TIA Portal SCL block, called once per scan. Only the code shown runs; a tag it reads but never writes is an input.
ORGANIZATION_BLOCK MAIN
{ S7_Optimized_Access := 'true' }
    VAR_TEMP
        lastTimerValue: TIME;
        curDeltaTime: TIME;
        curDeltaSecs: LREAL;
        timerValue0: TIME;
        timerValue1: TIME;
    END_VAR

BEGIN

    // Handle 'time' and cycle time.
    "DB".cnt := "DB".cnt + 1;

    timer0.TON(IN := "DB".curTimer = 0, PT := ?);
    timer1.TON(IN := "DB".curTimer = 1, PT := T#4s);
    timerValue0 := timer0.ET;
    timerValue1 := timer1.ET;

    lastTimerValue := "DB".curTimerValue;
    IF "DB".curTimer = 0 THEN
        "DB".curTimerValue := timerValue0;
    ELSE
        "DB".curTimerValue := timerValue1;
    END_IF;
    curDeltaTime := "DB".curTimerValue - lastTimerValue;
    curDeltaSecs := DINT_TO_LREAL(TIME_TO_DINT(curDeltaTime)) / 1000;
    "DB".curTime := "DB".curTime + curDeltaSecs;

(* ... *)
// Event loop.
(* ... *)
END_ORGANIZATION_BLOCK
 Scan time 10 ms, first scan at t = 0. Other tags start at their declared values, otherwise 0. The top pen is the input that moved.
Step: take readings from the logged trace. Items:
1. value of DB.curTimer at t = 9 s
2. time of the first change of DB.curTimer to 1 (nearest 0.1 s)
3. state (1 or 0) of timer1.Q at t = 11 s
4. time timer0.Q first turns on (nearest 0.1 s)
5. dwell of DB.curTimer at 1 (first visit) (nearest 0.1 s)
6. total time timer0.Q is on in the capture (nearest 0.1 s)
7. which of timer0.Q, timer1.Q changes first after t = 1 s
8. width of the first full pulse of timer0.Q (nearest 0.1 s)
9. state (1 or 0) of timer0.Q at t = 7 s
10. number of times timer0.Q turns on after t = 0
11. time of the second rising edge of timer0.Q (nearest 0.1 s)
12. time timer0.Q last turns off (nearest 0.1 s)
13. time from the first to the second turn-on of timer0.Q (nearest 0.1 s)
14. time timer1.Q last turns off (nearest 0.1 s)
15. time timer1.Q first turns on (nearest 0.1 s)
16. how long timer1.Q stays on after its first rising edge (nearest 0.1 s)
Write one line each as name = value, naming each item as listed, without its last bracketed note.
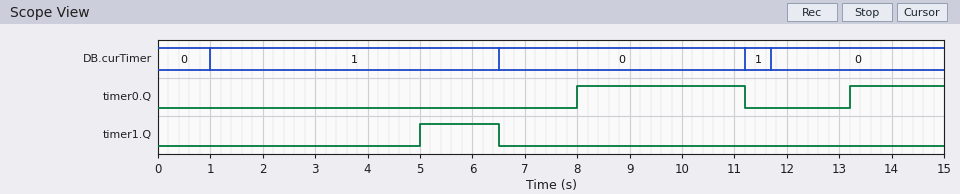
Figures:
value of DB.curTimer at t = 9 s = 0
time of the first change of DB.curTimer to 1 = 1.0 s
state (1 or 0) of timer1.Q at t = 11 s = 0
time timer0.Q first turns on = 8.0 s
dwell of DB.curTimer at 1 (first visit) = 5.5 s
total time timer0.Q is on in the capture = 5.0 s
which of timer0.Q, timer1.Q changes first after t = 1 s = timer1.Q
width of the first full pulse of timer0.Q = 3.2 s
state (1 or 0) of timer0.Q at t = 7 s = 0
number of times timer0.Q turns on after t = 0 = 2
time of the second rising edge of timer0.Q = 13.2 s
time timer0.Q last turns off = 11.2 s
time from the first to the second turn-on of timer0.Q = 5.2 s
time timer1.Q last turns off = 6.5 s
time timer1.Q first turns on = 5.0 s
how long timer1.Q stays on after its first rising edge = 1.5 s
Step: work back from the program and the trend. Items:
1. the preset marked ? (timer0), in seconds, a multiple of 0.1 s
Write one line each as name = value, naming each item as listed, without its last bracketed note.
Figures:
the preset marked ? (timer0), in seconds, a multiple of 0.1 s = 1.5 s
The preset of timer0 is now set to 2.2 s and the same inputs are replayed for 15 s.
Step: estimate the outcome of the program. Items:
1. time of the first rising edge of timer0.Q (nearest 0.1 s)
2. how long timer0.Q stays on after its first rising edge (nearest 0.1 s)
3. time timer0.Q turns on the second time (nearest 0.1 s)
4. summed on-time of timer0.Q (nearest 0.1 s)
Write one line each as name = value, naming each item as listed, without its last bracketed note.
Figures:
time of the first rising edge of timer0.Q = 8.7 s
how long timer0.Q stays on after its first rising edge = 2.5 s
time timer0.Q turns on the second time = 13.9 s
summed on-time of timer0.Q = 3.6 s
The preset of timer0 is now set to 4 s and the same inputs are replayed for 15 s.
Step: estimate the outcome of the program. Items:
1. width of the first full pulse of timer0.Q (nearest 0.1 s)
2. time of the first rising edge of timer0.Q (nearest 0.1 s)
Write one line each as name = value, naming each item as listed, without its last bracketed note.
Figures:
width of the first full pulse of timer0.Q = 0.7 s
time of the first rising edge of timer0.Q = 10.5 s
